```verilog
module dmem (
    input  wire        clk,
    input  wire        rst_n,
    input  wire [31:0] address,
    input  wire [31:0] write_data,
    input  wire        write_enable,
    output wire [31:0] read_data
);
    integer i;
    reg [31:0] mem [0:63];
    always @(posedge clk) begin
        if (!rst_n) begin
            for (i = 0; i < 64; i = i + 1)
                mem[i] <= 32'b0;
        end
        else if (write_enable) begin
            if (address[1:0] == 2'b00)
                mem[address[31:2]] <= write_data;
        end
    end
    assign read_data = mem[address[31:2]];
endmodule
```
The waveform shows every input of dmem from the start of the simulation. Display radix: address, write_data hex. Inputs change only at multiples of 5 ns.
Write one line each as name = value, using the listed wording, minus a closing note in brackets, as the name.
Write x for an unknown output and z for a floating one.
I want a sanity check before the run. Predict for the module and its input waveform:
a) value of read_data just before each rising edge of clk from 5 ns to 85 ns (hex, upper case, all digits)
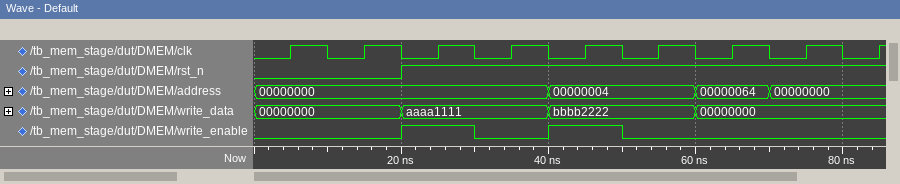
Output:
value of read_data just before each rising edge of clk from 5 ns to 85 ns = x, 00000000, 00000000, AAAA1111, 00000000, BBBB2222, 00000000, AAAA1111, AAAA1111
